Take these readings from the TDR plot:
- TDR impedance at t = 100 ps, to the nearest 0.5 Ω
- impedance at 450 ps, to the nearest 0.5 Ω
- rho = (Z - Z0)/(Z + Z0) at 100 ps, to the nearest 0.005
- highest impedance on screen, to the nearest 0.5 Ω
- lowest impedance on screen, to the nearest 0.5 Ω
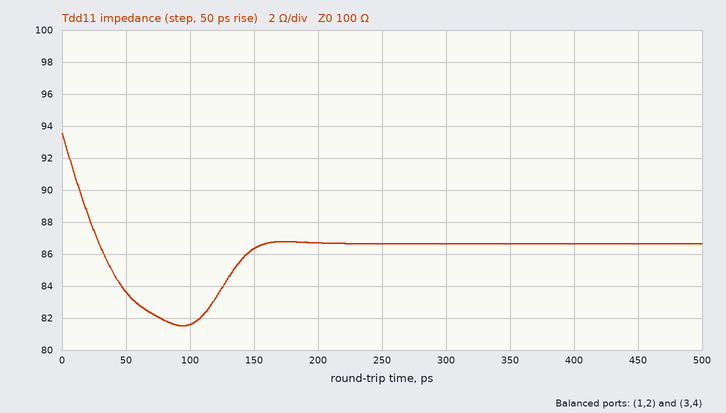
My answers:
81.5 Ω
86.5 Ω
-0.100
93.5 Ω
81.5 Ω
